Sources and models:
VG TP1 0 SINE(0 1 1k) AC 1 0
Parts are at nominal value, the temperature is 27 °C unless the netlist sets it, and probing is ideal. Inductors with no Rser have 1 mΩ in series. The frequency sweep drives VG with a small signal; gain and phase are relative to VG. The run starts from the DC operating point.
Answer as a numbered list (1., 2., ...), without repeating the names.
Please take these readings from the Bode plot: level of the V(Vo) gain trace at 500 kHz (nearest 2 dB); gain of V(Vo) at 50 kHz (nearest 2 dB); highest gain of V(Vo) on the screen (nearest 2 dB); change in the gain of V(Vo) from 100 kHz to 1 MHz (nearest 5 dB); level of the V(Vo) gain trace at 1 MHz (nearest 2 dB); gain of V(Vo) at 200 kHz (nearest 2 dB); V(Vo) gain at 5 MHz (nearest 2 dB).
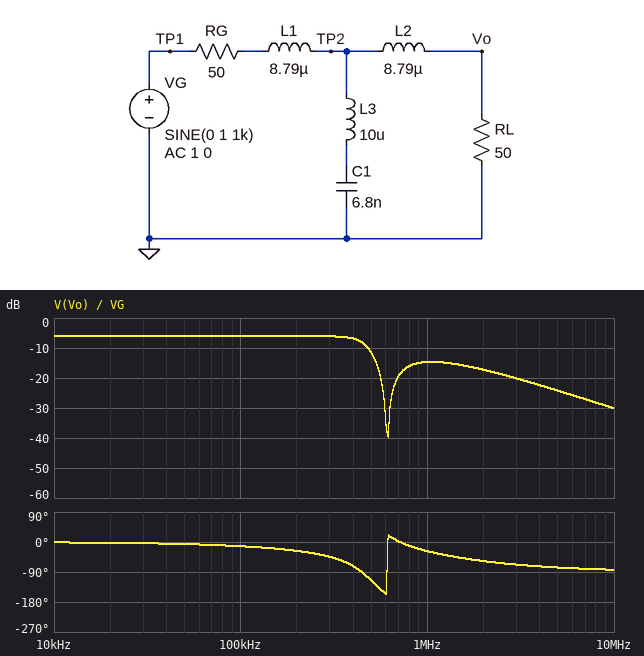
1. -12 dB
2. -6 dB
3. -6 dB
4. -10 dB
5. -14 dB
6. -6 dB
7. -24 dB
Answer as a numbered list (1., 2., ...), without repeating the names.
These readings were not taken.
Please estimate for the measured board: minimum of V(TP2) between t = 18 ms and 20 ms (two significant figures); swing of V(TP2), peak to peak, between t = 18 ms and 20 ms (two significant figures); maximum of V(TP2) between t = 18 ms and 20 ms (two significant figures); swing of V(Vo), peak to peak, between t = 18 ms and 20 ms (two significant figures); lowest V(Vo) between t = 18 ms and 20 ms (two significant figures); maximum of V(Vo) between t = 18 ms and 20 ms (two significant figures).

1. -500 mV
2. 1.0 V
3. 500 mV
4. 1.0 V
5. -500 mV
6. 500 mV
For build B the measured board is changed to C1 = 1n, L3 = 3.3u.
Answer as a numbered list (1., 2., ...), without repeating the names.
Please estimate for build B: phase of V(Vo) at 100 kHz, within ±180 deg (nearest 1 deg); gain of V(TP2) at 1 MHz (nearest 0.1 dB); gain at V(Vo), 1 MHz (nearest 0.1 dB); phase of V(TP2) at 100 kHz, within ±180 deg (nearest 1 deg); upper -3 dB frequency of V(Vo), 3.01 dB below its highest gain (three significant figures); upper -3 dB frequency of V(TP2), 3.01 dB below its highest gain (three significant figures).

1. -7 deg
2. -4.3 dB
3. -7.8 dB
4. -1 deg
5. 1.91 MHz
6. 1.94 MHz
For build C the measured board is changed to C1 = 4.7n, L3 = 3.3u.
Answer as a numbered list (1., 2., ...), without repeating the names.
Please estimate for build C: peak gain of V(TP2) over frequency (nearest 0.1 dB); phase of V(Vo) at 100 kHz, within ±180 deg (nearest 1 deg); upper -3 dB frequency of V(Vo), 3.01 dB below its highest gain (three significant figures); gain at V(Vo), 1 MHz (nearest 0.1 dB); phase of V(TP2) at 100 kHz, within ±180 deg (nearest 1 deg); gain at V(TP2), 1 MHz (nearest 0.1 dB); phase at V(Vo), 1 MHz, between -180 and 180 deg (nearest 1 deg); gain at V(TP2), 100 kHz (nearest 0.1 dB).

1. -4.5 dB
2. -11 deg
3. 825 kHz
4. -16.3 dB
5. -4 deg
6. -12.9 dB
7. -168 deg
8. -6.0 dB
